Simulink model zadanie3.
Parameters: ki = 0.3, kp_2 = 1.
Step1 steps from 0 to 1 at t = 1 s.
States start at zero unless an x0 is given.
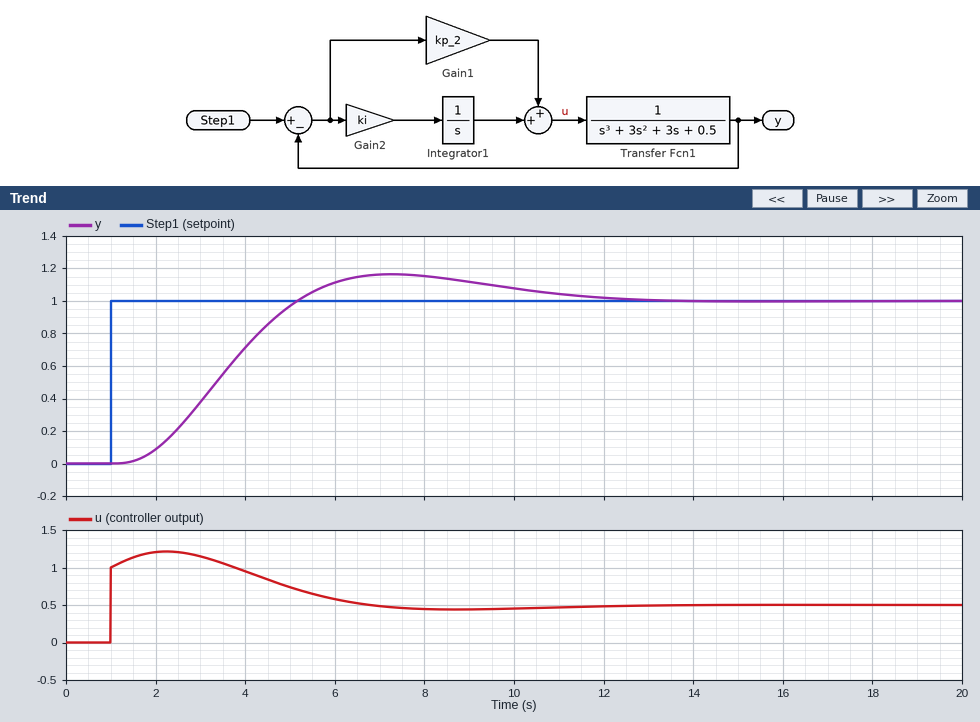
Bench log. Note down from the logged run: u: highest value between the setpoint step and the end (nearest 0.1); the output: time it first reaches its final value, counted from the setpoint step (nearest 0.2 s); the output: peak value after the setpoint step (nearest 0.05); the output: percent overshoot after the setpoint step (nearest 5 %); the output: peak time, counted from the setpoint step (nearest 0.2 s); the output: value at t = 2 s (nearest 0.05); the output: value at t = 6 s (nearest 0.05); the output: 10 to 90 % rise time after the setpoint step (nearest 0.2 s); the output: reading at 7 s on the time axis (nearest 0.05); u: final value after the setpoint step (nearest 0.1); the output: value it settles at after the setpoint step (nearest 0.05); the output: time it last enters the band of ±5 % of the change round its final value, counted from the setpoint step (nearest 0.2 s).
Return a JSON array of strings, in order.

["1.2", "4.2 s", "1.15", "15 %", "6.2 s", "0.10", "1.10", "2.6 s", "1.15", "0.5", "1.00", "9.8 s"]
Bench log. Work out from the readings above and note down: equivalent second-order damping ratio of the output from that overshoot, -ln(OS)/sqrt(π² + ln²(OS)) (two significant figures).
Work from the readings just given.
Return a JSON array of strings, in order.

["0.52"]
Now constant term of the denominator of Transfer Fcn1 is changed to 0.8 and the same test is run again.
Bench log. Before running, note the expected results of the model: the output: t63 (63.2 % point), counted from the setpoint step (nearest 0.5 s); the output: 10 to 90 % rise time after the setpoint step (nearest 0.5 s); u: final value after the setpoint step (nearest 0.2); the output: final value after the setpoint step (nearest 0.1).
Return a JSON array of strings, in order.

["3.0 s", "3.0 s", "0.8", "1.0"]
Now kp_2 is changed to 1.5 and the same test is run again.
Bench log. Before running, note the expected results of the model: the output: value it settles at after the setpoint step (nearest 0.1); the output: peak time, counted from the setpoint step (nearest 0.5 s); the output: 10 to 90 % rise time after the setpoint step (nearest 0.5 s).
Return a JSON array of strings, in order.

["1.0", "4.5 s", "2.0 s"]
